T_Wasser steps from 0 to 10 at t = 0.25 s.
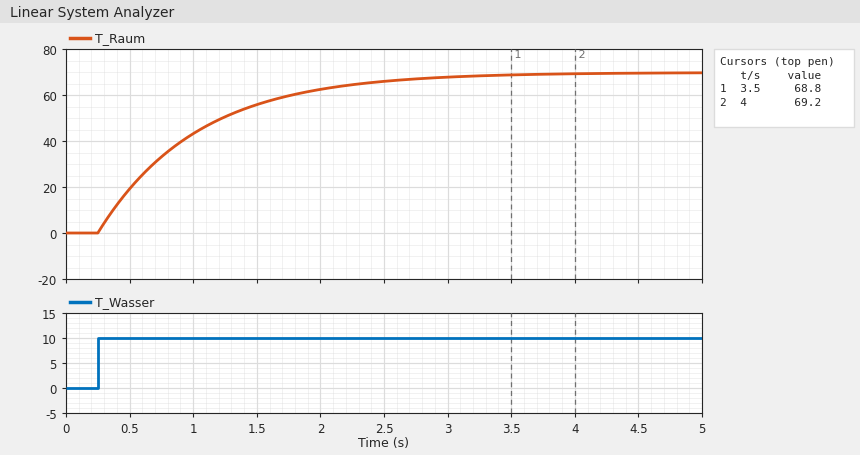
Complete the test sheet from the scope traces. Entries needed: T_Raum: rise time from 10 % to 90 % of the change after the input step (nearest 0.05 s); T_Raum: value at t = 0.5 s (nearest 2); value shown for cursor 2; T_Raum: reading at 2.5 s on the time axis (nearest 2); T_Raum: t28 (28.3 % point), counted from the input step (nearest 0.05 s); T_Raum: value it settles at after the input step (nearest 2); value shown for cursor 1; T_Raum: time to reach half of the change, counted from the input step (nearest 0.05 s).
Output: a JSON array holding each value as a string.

["1.70 s", "20", "69.2", "66", "0.25 s", "70", "68.8", "0.55 s"]
